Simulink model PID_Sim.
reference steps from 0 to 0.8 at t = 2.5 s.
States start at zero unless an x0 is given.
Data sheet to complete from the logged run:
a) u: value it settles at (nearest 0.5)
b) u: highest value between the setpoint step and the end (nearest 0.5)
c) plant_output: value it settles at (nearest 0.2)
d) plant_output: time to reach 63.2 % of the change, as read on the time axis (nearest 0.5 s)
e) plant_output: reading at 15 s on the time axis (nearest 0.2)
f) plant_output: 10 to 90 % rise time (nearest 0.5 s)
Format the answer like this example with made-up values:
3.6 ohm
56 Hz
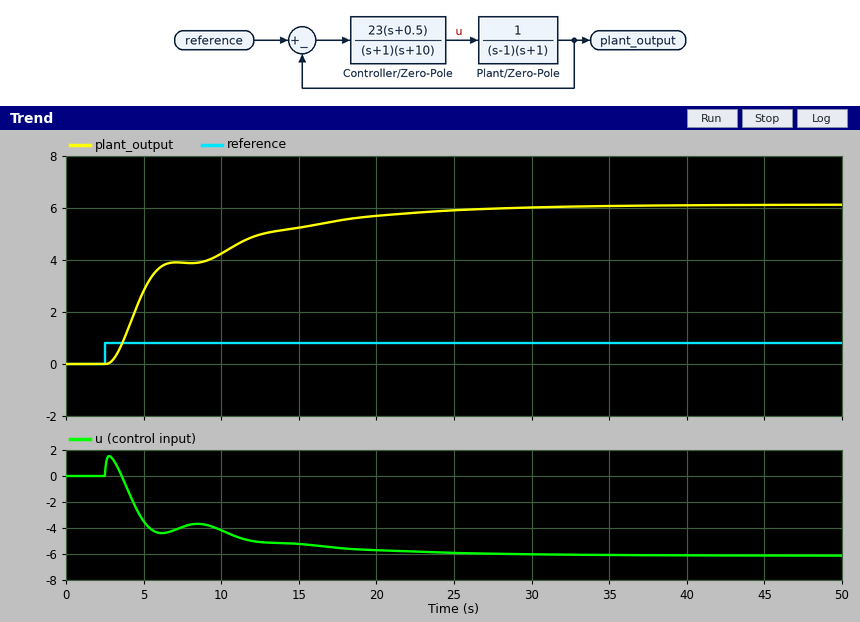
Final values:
-6.0
1.5
6.2
6.5 s
5.2
14.0 s
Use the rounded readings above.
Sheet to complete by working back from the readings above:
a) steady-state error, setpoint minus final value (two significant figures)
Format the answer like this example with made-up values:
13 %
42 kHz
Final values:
-5.4
